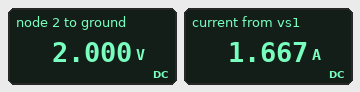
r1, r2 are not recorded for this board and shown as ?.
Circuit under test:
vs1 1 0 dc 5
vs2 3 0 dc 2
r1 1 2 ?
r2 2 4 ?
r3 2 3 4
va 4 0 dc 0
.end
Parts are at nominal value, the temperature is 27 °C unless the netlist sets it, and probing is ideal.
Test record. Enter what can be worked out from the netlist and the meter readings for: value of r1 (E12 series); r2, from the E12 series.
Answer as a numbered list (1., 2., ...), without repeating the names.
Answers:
1. 1.8 Ω
2. 1.2 Ω
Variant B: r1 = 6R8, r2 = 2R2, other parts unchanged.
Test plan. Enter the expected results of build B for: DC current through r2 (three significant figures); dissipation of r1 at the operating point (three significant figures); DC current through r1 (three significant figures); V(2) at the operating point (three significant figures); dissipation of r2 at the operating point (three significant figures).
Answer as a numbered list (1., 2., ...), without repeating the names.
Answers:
1. 659 mA
2. 1.85 W
3. 522 mA
4. 1.45 V
5. 956 mW
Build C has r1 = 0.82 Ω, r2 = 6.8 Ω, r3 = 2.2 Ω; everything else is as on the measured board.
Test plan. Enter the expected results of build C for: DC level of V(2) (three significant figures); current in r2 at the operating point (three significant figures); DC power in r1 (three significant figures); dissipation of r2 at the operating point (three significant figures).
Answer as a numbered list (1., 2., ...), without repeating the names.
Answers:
1. 3.85 V
2. 566 mA
3. 1.62 W
4. 2.18 W
